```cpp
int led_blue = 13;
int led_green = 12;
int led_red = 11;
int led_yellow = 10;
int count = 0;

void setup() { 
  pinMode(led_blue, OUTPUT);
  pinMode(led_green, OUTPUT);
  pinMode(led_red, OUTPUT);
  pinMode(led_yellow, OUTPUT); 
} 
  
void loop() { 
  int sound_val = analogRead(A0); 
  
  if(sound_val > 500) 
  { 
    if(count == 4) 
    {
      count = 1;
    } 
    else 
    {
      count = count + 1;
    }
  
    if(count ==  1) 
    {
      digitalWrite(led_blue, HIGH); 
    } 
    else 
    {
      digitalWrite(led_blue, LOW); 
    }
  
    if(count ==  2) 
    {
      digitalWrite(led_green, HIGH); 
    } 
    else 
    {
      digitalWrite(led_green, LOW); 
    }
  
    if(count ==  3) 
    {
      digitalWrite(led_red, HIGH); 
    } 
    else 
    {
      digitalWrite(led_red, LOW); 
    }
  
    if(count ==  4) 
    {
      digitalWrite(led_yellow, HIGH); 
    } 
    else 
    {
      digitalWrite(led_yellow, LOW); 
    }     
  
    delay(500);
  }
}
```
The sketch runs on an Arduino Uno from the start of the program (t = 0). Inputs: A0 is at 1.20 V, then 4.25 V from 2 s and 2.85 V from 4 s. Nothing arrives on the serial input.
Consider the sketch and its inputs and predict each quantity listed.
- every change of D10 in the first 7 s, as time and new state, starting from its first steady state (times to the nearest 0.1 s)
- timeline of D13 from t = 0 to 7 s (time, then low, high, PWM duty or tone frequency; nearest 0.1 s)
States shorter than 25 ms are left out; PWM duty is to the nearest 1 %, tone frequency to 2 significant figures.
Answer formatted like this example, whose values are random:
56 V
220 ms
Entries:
0 s low; 3.5 s high; 4 s low; 5.5 s high; 6 s low
0 s low; 2 s high; 2.5 s low; 4 s high; 4.5 s low; 6 s high; 6.5 s low
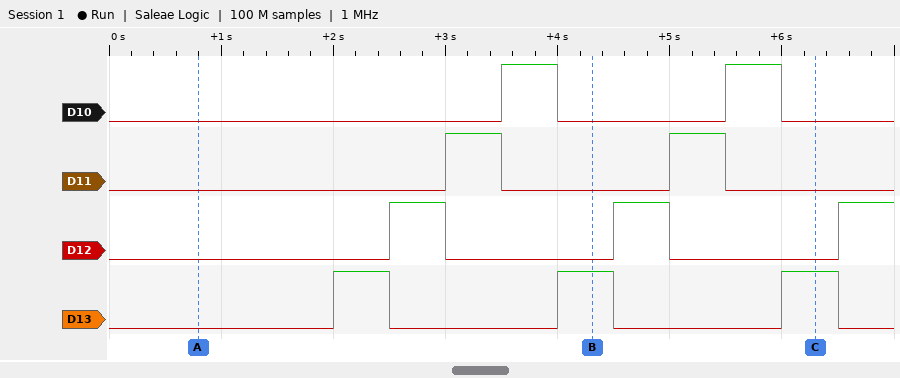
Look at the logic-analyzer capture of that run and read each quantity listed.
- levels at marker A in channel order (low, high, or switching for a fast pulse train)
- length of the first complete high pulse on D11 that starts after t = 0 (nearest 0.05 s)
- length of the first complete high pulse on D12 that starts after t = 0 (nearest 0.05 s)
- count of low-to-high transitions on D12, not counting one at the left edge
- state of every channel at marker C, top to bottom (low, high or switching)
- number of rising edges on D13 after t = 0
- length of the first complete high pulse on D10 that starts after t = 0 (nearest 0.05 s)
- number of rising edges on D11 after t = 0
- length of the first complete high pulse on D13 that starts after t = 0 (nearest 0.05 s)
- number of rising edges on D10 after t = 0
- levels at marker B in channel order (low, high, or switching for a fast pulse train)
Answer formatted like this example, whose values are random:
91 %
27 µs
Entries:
D10 low, D11 low, D12 low, D13 low
0.50 s
0.50 s
3
D10 low, D11 low, D12 low, D13 high
3
0.50 s
2
0.50 s
2
D10 low, D11 low, D12 low, D13 high
